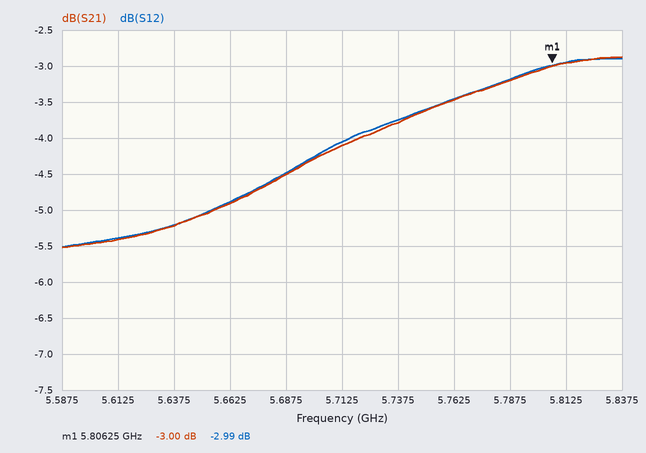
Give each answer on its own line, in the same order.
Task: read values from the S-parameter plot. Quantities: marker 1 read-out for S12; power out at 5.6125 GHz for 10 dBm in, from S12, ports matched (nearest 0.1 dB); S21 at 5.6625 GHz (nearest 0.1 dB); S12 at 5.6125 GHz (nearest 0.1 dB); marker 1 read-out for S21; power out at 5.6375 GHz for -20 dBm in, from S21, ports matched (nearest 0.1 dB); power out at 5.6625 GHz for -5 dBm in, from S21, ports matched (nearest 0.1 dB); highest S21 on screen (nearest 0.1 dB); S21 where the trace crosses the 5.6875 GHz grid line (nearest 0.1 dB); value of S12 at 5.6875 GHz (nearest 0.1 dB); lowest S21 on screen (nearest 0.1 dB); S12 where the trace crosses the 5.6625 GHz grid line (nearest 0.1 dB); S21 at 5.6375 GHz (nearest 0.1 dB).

-2.99 dB
4.6 dBm
-4.9 dB
-5.4 dB
-3.00 dB
-25.2 dBm
-9.9 dBm
-2.9 dB
-4.5 dB
-4.5 dB
-5.5 dB
-4.9 dB
-5.2 dB
